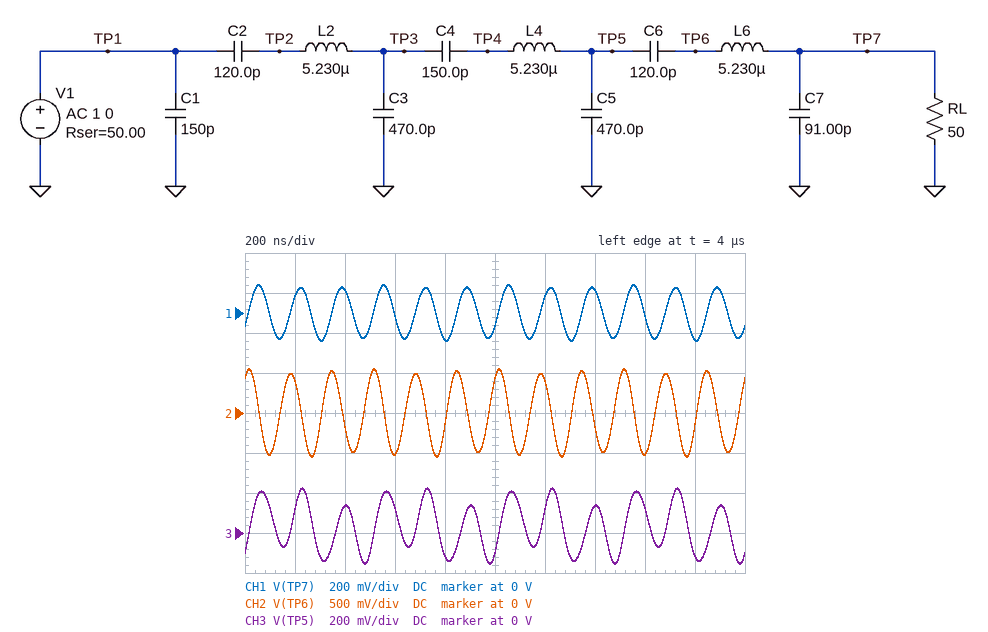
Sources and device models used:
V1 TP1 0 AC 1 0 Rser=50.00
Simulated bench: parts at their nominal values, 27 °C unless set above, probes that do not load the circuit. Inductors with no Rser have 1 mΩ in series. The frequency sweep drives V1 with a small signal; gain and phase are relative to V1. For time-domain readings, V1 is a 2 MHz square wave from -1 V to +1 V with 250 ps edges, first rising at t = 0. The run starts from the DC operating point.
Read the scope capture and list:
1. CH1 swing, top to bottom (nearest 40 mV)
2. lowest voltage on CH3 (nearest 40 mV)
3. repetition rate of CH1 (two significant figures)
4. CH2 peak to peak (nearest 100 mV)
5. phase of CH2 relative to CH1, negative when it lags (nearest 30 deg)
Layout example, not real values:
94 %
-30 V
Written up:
280 mV
-160 mV
6.0 MHz
1.1 V
90 deg
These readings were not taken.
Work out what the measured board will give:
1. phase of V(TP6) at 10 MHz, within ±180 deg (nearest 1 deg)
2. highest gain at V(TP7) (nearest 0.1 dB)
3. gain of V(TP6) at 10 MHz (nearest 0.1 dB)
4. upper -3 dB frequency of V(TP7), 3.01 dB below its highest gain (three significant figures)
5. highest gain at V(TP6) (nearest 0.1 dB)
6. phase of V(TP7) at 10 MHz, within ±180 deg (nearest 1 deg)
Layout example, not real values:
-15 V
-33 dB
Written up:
1 deg
-6.0 dB
-19.9 dB
8.30 MHz
8.3 dB
-96 deg
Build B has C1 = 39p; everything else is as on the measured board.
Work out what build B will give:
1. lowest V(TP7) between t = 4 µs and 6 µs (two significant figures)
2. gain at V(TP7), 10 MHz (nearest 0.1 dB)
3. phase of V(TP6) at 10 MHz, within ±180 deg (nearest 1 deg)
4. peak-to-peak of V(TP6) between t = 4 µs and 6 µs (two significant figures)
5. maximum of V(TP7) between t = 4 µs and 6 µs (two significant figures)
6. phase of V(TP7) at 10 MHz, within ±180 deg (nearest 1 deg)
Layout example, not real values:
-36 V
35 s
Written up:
-150 mV
-36.4 dB
21 deg
1.2 V
150 mV
-76 deg
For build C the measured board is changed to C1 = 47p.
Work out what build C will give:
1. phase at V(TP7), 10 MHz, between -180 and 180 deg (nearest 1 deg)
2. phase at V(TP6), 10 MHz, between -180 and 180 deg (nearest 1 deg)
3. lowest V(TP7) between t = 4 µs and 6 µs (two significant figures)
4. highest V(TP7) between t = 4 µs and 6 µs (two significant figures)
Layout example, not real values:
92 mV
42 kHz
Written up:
-78 deg
20 deg
-150 mV
150 mV
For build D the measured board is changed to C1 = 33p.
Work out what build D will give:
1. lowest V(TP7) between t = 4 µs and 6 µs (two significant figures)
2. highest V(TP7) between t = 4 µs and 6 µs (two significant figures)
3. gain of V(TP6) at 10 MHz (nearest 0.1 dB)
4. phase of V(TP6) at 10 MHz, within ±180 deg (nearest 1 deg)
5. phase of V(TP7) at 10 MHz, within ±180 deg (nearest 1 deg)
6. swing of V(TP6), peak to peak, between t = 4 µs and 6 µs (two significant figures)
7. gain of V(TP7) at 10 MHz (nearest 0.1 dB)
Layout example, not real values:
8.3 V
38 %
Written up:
-150 mV
150 mV
-20.0 dB
22 deg
-75 deg
1.2 V
-36.4 dB
